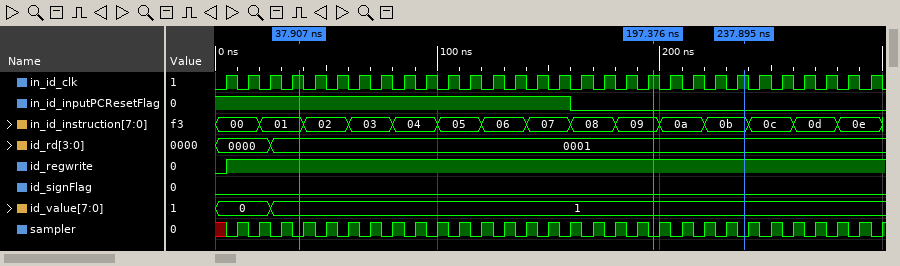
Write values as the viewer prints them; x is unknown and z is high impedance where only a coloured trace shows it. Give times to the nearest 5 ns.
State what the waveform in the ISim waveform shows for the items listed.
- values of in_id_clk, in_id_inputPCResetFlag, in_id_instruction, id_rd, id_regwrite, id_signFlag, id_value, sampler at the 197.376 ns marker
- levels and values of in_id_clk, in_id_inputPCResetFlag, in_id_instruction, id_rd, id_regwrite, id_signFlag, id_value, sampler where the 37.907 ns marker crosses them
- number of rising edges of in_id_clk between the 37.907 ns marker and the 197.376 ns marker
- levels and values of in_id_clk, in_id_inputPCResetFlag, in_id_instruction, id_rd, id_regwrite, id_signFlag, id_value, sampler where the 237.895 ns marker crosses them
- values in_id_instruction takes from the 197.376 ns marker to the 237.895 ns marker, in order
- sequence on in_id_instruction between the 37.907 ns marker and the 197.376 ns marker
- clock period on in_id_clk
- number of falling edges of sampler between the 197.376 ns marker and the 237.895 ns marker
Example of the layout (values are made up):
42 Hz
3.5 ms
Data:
in_id_clk=1, in_id_inputPCResetFlag=0, in_id_instruction=09, id_rd=0001, id_regwrite=1, id_signFlag=0, id_value=1, sampler=0
in_id_clk=1, in_id_inputPCResetFlag=1, in_id_instruction=01, id_rd=0001, id_regwrite=1, id_signFlag=0, id_value=1, sampler=0
16
in_id_clk=1, in_id_inputPCResetFlag=0, in_id_instruction=0b, id_rd=0001, id_regwrite=1, id_signFlag=0, id_value=1, sampler=0
09, 0a, 0b
01, 02, 03, 04, 05, 06, 07, 08, 09
10 ns
4
